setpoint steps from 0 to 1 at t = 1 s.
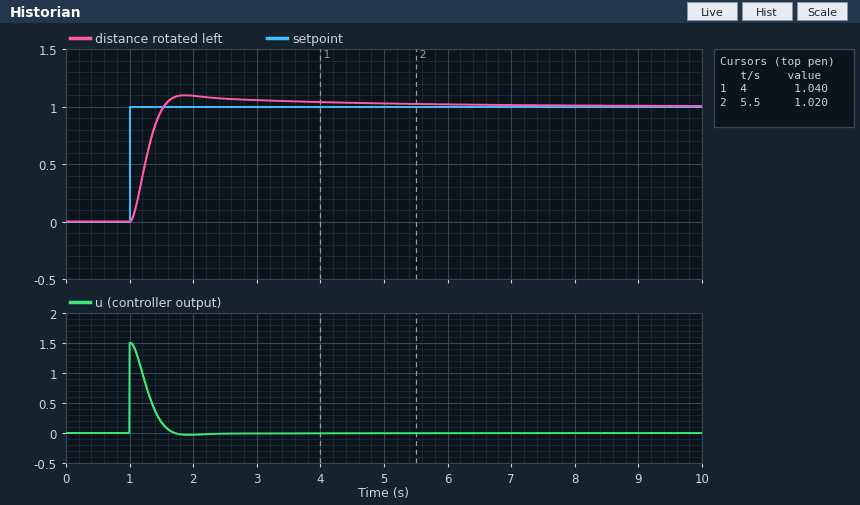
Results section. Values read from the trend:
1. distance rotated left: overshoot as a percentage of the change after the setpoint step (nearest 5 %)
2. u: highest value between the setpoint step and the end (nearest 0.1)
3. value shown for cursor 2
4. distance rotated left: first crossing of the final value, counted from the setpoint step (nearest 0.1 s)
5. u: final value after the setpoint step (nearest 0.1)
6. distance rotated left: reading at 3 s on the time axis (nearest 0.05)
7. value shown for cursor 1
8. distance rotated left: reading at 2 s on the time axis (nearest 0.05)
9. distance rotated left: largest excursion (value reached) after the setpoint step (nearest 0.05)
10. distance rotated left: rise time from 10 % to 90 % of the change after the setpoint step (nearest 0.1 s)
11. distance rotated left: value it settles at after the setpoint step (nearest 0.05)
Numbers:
10 %
1.5
1.020
0.5 s
0.0
1.05
1.040
1.10
1.10
0.4 s
1.00
